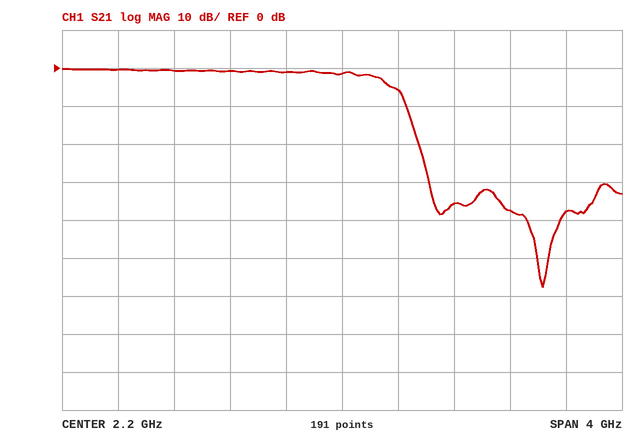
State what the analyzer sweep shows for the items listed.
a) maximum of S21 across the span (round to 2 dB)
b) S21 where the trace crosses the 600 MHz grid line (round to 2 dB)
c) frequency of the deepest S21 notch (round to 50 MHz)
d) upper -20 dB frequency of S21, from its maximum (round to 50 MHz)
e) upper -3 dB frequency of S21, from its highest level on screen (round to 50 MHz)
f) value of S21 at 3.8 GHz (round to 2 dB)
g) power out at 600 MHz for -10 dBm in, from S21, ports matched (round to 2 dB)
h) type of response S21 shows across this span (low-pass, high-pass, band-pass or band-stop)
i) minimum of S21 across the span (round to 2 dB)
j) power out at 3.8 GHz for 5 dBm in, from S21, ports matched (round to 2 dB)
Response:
0 dB
0 dB
3.65 GHz
2.75 GHz
2.50 GHz
-38 dB
-10 dBm
low-pass
-58 dB
-32 dBm
